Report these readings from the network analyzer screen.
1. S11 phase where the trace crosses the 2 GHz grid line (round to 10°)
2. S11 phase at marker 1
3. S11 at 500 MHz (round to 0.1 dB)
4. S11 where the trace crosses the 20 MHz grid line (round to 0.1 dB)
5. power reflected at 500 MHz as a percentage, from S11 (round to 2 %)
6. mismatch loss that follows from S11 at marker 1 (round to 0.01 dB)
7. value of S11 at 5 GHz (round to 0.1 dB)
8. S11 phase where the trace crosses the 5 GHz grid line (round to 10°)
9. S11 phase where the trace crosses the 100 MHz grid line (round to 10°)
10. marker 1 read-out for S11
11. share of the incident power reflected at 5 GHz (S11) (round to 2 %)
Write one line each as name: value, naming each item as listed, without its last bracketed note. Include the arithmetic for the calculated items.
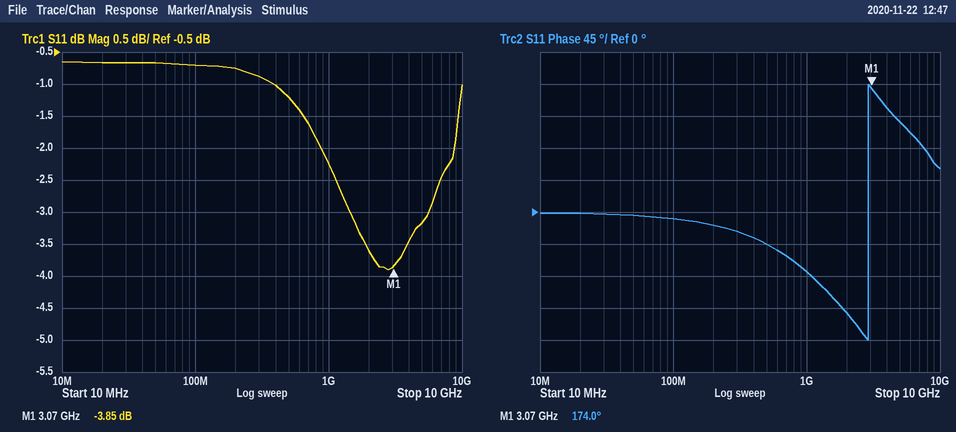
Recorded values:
S11 phase where the trace crosses the 2 GHz grid line: -140°
S11 phase at marker 1: 174.0°
S11 at 500 MHz: -1.2 dB
S11 where the trace crosses the 20 MHz grid line: -0.7 dB
power reflected at 500 MHz as a percentage, from S11: 10^(-1.2/10) ≈ 76 %
mismatch loss that follows from S11 at marker 1: −10 log10(1 − 10^(-3.85/10)) ≈ 2.31 dB
value of S11 at 5 GHz: -3.2 dB
S11 phase where the trace crosses the 5 GHz grid line: 130°
S11 phase where the trace crosses the 100 MHz grid line: -10°
marker 1 read-out for S11: -3.85 dB
share of the incident power reflected at 5 GHz (S11): 10^(-3.2/10) ≈ 48 %
